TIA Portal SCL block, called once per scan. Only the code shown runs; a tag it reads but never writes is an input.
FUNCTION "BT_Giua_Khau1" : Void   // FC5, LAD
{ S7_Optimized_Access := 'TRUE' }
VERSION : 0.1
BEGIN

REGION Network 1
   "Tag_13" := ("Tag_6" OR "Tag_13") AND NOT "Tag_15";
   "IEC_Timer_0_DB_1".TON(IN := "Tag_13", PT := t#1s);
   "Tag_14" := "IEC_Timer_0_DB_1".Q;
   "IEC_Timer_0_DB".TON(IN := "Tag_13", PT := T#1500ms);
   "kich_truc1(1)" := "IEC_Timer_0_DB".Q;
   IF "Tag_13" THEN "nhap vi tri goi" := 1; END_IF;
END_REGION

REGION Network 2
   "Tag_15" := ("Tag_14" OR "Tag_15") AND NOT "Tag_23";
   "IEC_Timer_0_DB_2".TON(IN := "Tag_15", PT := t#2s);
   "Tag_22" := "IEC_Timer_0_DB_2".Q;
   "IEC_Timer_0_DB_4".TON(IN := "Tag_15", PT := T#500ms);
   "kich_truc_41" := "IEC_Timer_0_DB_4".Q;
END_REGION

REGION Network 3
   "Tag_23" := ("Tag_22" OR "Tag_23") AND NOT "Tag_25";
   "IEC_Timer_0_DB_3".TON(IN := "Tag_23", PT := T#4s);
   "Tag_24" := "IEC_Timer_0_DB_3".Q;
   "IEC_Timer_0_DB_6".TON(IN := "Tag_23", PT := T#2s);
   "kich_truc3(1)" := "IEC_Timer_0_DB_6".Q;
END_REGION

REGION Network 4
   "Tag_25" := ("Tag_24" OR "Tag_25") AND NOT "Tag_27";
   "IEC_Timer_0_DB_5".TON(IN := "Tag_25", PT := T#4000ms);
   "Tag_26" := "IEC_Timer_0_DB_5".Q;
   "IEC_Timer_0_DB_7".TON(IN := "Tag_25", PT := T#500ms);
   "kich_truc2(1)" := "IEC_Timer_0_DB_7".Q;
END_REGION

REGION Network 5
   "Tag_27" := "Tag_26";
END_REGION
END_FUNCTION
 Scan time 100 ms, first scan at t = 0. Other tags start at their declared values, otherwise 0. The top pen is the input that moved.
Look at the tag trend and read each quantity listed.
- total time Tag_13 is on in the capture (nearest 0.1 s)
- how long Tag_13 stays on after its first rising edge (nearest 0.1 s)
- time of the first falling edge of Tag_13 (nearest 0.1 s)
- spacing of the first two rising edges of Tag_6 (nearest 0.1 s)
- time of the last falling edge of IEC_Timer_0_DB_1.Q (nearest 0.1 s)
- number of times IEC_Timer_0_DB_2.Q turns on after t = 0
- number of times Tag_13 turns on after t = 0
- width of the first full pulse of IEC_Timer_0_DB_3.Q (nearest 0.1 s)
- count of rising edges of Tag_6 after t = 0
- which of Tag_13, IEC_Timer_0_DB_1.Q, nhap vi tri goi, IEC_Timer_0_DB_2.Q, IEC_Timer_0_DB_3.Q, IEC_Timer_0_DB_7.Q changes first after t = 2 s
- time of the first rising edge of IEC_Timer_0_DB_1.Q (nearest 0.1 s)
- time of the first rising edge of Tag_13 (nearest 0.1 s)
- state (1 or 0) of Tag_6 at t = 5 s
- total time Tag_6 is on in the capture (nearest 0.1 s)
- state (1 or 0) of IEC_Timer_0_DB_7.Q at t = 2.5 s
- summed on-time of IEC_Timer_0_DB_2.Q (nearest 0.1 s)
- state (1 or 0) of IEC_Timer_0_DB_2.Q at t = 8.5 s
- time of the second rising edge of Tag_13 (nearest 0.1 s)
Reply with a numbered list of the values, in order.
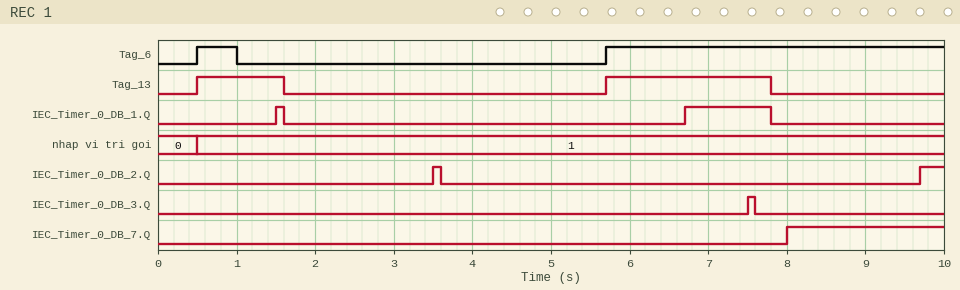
1. 3.2 s
2. 1.1 s
3. 1.6 s
4. 5.2 s
5. 7.8 s
6. 2
7. 2
8. 0.1 s
9. 2
10. IEC_Timer_0_DB_2.Q
11. 1.5 s
12. 0.5 s
13. 0
14. 4.8 s
15. 0
16. 0.4 s
17. 0
18. 5.7 s
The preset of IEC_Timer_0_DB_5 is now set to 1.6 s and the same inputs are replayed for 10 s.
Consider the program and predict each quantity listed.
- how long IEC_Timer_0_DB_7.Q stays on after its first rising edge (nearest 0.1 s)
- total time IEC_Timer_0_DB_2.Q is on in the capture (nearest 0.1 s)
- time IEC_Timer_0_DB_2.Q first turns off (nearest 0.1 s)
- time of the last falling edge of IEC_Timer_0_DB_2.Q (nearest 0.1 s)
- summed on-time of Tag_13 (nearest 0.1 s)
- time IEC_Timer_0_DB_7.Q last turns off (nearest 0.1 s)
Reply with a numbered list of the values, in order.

1. 1.2 s
2. 0.2 s
3. 3.6 s
4. 9.8 s
5. 3.3 s
6. 9.2 s
